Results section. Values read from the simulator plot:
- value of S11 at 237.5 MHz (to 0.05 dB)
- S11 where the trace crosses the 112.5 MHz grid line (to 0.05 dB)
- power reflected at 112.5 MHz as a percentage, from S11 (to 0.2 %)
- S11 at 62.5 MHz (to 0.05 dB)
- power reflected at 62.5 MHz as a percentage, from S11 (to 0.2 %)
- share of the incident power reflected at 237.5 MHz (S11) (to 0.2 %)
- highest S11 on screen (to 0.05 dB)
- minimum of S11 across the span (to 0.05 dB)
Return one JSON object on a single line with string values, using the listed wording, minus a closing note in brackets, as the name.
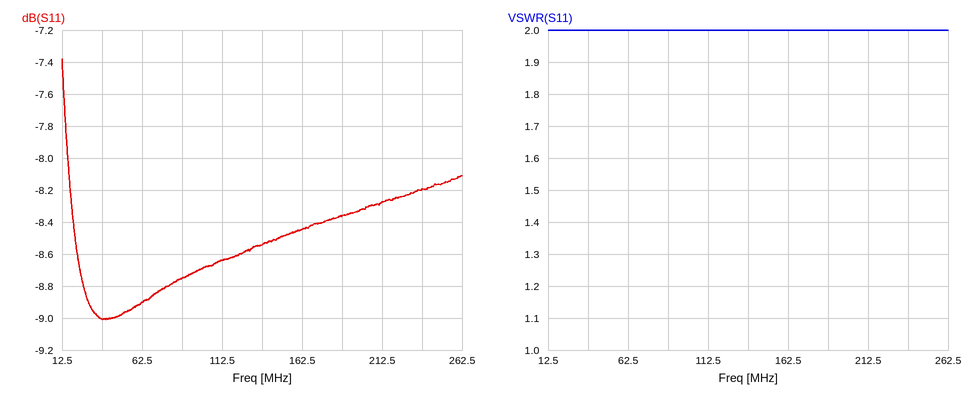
{"value of S11 at 237.5 MHz": "-8.20 dB", "S11 where the trace crosses the 112.5 MHz grid line": "-8.65 dB", "power reflected at 112.5 MHz as a percentage, from S11": "13.6 %", "S11 at 62.5 MHz": "-8.90 dB", "power reflected at 62.5 MHz as a percentage, from S11": "12.8 %", "share of the incident power reflected at 237.5 MHz (S11)": "15.2 %", "highest S11 on screen": "-7.40 dB", "minimum of S11 across the span": "-9.00 dB"}
